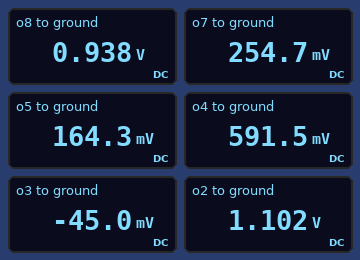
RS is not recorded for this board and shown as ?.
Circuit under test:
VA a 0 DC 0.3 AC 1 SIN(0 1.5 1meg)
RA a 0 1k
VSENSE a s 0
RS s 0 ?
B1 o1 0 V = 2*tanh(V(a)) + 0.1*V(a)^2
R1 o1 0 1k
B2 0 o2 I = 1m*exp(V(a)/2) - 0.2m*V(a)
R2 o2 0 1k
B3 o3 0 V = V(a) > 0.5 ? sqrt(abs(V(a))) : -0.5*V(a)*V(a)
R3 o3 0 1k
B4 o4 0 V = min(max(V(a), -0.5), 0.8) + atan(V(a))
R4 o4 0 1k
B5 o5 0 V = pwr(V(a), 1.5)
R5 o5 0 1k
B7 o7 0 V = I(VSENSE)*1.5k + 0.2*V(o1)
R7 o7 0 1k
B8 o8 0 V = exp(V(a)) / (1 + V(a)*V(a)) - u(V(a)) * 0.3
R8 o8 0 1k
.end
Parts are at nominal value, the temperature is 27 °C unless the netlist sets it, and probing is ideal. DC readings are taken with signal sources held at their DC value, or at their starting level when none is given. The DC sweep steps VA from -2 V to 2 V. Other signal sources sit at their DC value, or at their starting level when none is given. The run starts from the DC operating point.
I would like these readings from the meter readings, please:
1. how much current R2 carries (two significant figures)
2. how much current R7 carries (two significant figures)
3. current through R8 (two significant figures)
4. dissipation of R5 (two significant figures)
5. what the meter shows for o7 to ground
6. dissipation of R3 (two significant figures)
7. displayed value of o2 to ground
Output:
1.1 mA
250 µA
940 µA
27 µW
254.7 mV
2.0 µW
1.102 V
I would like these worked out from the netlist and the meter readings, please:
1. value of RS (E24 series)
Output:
3.3 kΩ
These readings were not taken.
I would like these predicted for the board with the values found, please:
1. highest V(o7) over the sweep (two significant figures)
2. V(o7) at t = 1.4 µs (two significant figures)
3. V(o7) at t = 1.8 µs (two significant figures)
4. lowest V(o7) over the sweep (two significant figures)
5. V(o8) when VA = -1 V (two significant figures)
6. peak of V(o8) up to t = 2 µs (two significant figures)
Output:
1.4 V
700 mV
-960 mV
-1.2 V
180 mV
1.1 V
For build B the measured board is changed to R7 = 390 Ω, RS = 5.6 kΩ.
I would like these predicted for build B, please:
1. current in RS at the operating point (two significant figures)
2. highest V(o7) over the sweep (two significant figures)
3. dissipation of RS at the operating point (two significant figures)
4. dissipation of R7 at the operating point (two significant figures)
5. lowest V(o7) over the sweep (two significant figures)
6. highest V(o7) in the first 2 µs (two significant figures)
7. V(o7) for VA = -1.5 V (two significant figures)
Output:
54 µA
1.0 V
16 µW
100 µW
-840 mV
810 mV
-720 mV
